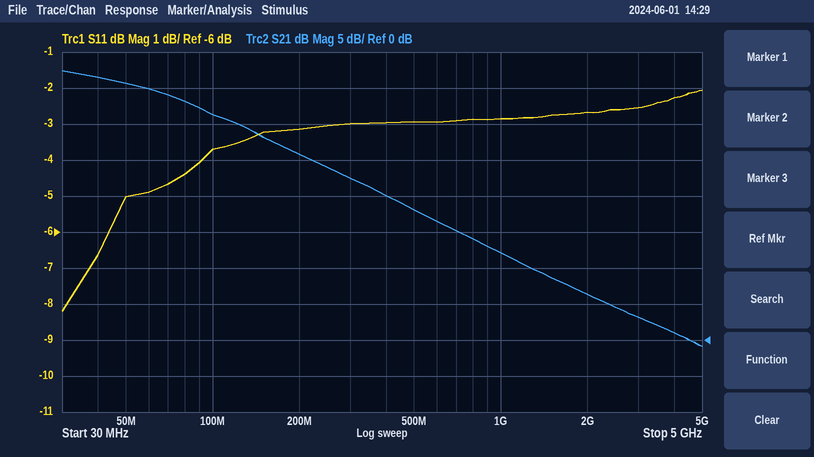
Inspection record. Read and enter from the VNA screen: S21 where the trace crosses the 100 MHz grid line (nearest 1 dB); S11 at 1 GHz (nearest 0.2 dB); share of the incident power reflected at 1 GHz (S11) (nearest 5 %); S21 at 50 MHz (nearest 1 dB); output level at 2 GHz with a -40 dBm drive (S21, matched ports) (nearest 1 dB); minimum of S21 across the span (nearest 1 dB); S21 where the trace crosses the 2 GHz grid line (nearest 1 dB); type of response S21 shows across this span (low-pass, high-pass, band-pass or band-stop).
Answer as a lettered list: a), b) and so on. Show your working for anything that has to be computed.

a) 31 dB
b) -2.8 dB
c) 10^(-2.8/10) ≈ 52.5 %, so 50 % to the nearest 5 %
d) 36 dB
e) -40 dBm + (6 dB) = -34 dBm
f) -1 dB
g) 6 dB
h) low-pass
